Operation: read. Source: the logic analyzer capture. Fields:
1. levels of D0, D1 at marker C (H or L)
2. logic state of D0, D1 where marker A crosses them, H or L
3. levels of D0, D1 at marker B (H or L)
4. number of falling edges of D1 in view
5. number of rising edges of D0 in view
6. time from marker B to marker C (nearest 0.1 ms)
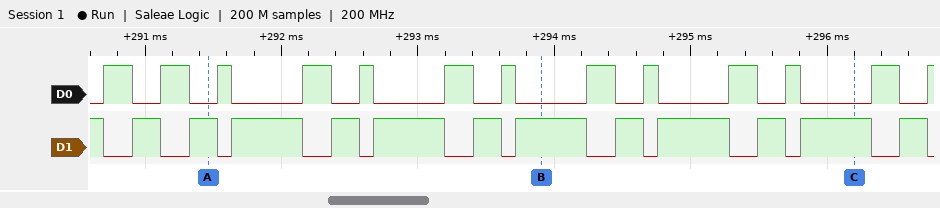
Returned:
D0=L, D1=H
D0=L, D1=H
D0=L, D1=H
13
13
2.3 ms
